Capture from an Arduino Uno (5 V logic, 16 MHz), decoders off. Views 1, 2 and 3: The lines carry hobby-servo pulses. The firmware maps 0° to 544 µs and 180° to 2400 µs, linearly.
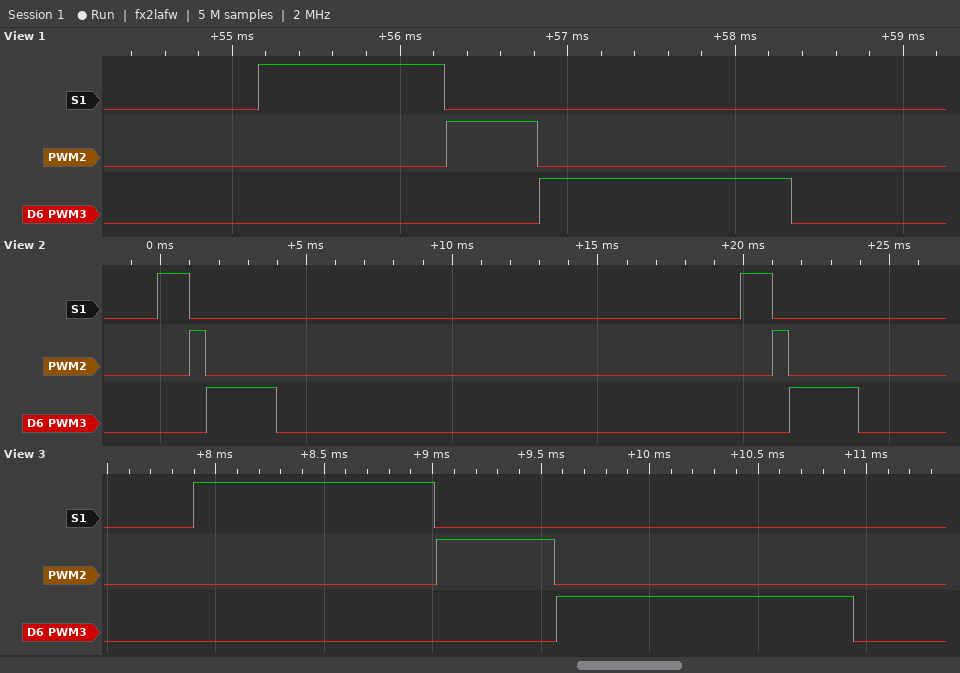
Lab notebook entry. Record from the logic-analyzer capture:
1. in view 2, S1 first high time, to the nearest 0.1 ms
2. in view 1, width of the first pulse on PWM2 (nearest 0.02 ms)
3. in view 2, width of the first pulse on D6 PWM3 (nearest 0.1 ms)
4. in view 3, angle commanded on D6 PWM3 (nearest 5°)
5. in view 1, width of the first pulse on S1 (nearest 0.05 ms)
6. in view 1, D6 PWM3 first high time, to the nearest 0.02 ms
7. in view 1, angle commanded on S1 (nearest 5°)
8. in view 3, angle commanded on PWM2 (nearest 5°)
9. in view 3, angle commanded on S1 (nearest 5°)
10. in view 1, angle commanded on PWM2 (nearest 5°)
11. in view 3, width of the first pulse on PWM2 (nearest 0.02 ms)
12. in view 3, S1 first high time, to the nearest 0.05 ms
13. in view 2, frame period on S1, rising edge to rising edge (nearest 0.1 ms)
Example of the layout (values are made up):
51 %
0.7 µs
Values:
1.1 ms
0.54 ms
2.4 ms
80°
1.10 ms
1.50 ms
55°
0°
55°
0°
0.54 ms
1.10 ms
20.0 ms
